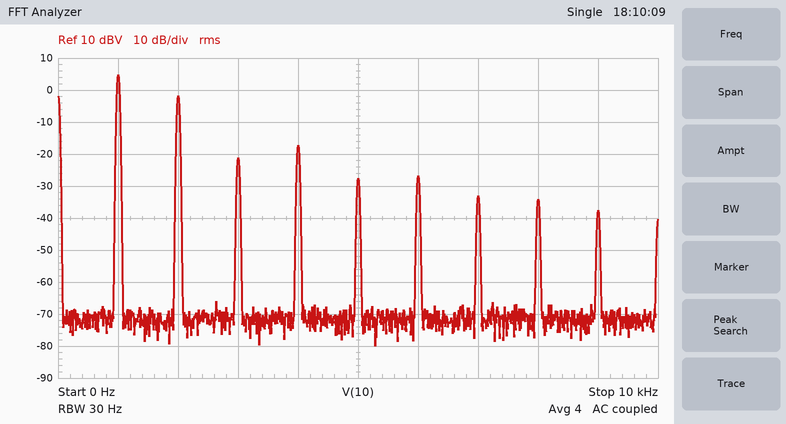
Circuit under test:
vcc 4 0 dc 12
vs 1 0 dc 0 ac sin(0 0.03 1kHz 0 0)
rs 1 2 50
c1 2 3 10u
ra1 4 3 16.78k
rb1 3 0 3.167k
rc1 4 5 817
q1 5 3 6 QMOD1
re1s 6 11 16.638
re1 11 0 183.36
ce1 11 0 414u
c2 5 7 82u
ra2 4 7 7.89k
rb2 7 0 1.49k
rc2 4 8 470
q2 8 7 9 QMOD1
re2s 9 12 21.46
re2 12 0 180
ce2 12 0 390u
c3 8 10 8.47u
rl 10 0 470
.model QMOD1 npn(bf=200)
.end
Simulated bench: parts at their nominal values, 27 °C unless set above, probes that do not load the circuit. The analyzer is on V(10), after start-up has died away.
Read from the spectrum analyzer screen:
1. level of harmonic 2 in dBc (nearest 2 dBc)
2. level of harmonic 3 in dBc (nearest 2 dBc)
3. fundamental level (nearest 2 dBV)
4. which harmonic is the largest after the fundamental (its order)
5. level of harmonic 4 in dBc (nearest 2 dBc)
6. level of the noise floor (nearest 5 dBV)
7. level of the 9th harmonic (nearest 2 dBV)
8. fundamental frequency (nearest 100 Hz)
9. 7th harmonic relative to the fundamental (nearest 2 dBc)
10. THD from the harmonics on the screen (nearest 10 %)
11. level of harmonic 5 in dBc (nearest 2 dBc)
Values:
-6 dBc
-26 dBc
4 dBV
2
-22 dBc
-70 dBV
-38 dBV
1.0 kHz
-38 dBc
50 %
-32 dBc
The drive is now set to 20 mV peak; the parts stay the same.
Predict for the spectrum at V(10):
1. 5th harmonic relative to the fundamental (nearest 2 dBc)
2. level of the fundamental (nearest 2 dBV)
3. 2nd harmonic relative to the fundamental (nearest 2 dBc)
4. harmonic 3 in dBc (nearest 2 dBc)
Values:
-36 dBc
4 dBV
-8 dBc
-32 dBc
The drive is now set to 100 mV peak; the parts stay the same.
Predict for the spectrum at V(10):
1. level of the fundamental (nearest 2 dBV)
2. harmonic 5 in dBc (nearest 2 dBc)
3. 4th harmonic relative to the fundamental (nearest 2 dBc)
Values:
8 dBV
-16 dBc
-14 dBc
